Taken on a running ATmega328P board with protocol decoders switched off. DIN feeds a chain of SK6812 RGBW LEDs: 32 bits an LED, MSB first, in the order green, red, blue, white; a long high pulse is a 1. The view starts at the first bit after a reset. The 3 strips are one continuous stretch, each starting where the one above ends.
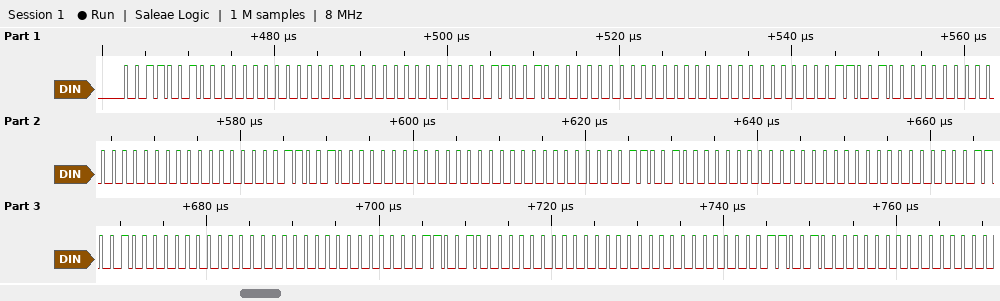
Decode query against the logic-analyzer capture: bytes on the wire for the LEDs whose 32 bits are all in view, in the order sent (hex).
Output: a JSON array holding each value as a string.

["32 00 00 00 32 00 00 00 32 00 00 00 32 00 00 00 32 00 00 00 32 00 00 00 32 00 00 00"]
